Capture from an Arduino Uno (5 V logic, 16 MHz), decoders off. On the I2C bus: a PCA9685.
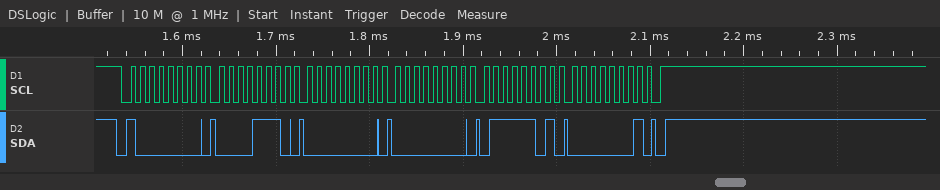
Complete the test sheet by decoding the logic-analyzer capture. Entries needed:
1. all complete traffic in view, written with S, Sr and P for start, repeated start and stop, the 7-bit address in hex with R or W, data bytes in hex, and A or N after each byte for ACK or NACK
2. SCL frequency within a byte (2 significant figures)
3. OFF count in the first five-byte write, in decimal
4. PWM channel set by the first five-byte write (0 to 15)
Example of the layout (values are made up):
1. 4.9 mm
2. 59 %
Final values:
1. S 40W A 0E A 00 A 00 A 7D A 01 A P
2. 100 kHz
3. 381
4. 2
